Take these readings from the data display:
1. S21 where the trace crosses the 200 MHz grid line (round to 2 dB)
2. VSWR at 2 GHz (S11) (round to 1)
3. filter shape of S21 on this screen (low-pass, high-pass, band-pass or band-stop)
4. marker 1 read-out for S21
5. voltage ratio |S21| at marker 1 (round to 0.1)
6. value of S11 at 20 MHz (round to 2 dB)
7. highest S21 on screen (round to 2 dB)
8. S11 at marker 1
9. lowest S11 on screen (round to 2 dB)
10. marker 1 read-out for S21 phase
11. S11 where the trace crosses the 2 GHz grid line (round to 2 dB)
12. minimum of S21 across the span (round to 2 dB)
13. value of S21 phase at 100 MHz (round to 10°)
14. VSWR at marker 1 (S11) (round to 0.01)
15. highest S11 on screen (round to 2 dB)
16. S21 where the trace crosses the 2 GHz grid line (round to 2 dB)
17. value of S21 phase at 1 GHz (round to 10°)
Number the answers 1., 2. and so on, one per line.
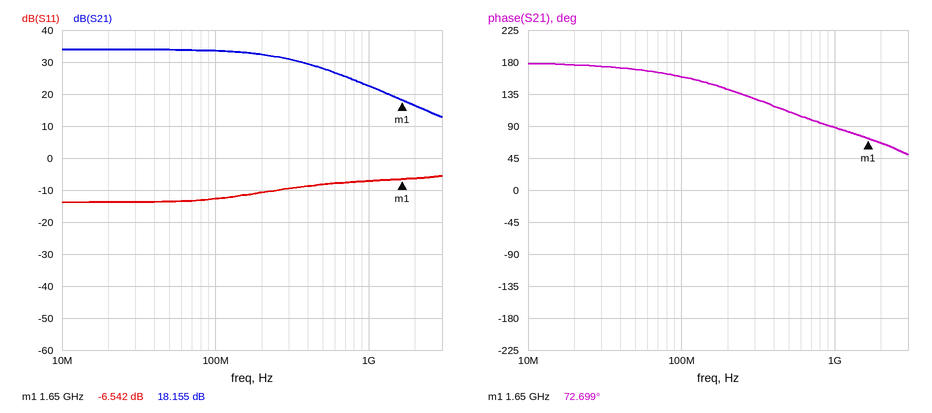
1. 32 dB
2. 3
3. low-pass
4. 18.155 dB
5. 8.1
6. -14 dB
7. 34 dB
8. -6.542 dB
9. -14 dB
10. 72.699°
11. -6 dB
12. 12 dB
13. 160°
14. 2.78
15. -6 dB
16. 16 dB
17. 90°
